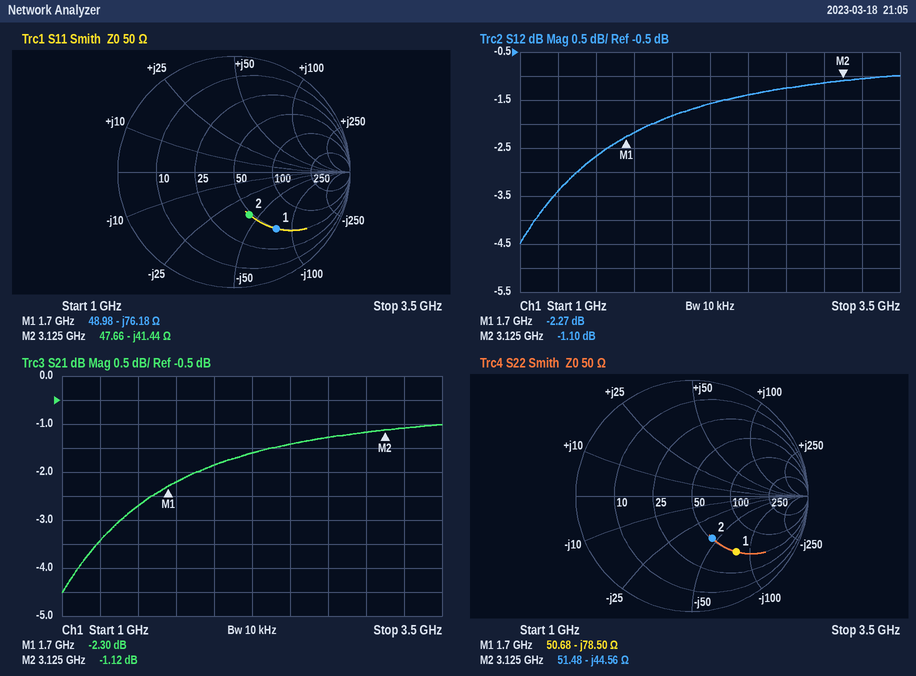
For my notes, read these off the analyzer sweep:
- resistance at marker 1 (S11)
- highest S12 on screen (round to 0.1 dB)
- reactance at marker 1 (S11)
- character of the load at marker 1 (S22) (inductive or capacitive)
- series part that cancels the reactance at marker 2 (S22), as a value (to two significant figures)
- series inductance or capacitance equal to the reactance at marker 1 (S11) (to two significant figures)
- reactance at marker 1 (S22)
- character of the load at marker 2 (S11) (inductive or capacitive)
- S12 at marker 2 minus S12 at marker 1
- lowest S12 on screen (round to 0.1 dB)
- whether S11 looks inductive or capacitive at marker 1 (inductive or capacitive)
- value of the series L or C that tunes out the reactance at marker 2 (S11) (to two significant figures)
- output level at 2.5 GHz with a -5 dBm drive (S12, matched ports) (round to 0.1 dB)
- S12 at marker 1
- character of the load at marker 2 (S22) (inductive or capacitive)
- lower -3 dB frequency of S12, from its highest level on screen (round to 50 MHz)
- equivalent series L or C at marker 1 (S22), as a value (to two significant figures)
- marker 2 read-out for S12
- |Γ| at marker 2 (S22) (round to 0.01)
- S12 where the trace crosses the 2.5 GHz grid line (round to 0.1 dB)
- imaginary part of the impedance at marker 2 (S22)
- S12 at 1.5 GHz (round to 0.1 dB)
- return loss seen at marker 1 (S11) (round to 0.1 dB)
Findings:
48.98 Ω
-1.0 dB
-76.18 Ω
capacitive
2.3 nH
1.2 pF
-78.50 Ω
capacitive
1.17 dB
-4.5 dB
capacitive
2.1 nH
-6.4 dBm
-2.27 dB
capacitive
1.10 GHz
1.2 pF
-1.10 dB
0.40
-1.4 dB
-44.56 Ω
-2.7 dB
4.3 dB
